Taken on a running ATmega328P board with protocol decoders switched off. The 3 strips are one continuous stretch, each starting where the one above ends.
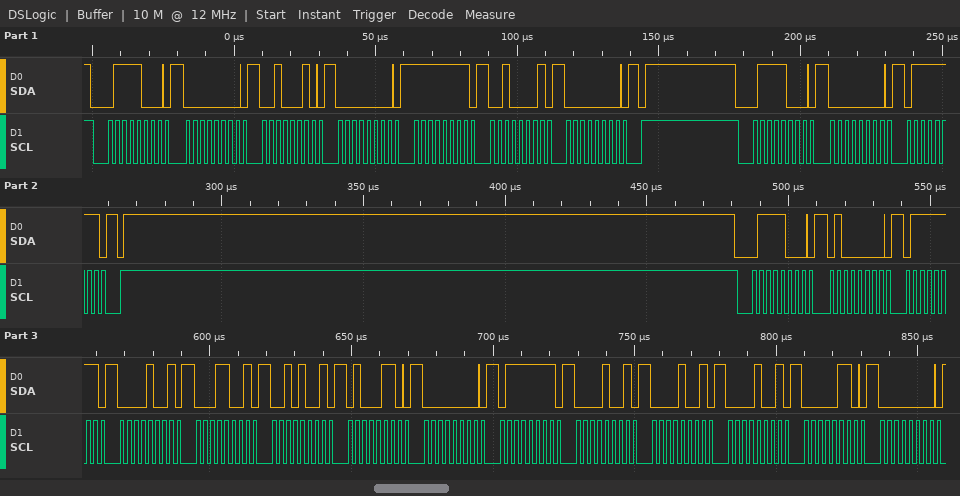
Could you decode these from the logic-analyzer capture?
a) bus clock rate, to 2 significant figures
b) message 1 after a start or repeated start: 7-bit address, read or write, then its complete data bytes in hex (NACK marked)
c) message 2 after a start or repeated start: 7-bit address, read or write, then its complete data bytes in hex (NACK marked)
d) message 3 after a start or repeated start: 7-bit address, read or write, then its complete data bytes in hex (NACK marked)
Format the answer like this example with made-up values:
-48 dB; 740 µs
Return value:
400 kHz; 0x3C write: 00 22 00 FF 21 00; 0x3C write: 00 7F; 0x3C write: 40 7F 09 19 29 46 00 7F 09 09 09 06 00
